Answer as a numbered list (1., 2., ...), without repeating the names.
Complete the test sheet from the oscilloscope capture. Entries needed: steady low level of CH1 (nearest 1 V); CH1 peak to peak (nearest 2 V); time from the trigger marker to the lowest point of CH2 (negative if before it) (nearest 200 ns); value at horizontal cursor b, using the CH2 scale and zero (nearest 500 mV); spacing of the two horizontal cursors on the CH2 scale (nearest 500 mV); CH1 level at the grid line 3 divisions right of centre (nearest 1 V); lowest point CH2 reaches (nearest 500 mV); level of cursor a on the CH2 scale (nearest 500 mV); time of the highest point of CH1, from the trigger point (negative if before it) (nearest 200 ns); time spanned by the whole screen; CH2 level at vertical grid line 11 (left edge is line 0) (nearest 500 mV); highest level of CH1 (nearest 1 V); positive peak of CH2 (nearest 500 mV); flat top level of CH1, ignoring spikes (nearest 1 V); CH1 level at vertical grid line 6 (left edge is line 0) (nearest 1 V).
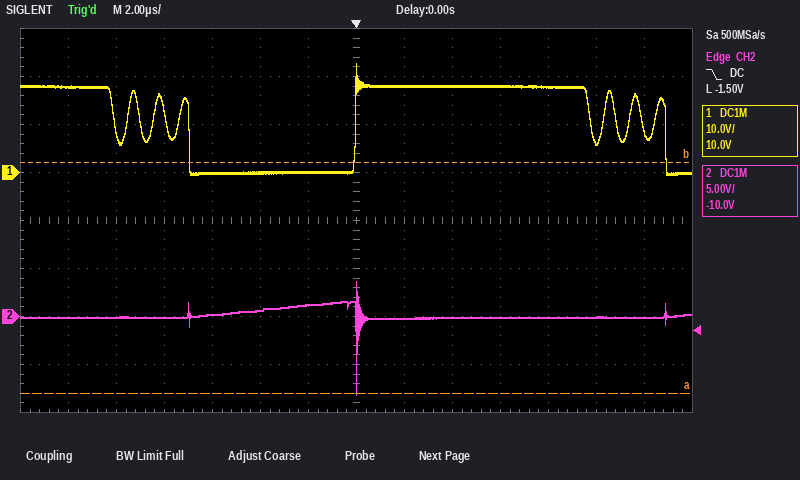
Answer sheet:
1. 0 V
2. 24 V
3. 0.0 µs
4. 16.0 V
5. 24.0 V
6. 18 V
7. -8.0 V
8. -8.0 V
9. 0.0 µs
10. 28 µs
11. 0.0 V
12. 23 V
13. 3.5 V
14. 18 V
15. 0 V
